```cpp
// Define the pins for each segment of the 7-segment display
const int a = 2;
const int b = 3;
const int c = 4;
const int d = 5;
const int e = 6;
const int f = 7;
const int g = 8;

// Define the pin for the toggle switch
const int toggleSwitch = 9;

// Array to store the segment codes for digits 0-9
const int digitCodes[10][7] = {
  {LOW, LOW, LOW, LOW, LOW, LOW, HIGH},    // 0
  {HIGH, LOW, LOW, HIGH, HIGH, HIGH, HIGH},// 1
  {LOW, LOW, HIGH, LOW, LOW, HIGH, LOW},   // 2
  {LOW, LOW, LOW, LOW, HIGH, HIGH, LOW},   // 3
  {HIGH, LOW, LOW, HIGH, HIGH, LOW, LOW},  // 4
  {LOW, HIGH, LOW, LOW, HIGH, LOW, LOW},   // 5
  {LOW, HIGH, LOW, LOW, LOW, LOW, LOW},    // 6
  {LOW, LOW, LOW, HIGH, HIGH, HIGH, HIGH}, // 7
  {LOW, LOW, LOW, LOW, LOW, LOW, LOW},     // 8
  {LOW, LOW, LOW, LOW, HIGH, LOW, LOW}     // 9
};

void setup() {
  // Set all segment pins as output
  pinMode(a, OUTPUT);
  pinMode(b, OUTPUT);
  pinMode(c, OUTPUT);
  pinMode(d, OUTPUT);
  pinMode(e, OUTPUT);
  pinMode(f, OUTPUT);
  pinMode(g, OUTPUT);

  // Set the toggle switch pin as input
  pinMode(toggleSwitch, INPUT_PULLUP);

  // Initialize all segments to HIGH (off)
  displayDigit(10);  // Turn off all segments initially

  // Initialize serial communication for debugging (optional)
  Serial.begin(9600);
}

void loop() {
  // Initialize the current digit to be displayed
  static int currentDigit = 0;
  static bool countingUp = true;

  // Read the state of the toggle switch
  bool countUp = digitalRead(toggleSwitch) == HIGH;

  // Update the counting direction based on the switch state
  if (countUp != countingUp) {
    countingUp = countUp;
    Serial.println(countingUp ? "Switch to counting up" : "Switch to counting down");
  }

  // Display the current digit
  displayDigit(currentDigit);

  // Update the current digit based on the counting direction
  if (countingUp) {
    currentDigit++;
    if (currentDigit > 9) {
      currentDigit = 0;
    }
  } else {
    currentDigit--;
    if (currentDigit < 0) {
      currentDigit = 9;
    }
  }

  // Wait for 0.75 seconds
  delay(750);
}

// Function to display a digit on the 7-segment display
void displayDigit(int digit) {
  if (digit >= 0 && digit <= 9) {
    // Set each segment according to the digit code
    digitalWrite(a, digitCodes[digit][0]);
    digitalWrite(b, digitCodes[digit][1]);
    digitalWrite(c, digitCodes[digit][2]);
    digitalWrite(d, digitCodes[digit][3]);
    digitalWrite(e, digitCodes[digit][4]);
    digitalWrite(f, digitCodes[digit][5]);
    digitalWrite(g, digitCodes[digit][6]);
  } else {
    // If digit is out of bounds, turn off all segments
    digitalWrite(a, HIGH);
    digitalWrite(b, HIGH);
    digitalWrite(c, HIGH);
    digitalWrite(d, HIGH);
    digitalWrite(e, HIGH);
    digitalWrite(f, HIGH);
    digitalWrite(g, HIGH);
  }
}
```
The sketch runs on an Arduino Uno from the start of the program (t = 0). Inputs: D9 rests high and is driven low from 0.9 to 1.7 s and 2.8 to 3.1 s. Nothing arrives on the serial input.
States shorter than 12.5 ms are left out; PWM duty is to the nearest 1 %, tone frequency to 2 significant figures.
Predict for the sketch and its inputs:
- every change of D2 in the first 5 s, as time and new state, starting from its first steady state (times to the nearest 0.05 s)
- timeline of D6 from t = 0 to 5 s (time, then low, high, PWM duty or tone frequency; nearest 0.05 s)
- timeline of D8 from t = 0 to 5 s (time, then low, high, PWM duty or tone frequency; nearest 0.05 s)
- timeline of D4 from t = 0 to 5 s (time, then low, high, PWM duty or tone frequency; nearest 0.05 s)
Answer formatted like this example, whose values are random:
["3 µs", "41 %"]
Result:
["0 s low; 0.75 s high; 1.5 s low; 2.25 s high; 3 s low; 3.75 s high; 4.5 s low", "0 s low; 0.75 s high; 1.5 s low; 2.25 s high; 3 s low; 3.75 s high; 4.5 s low", "0 s high; 1.5 s low; 2.25 s high; 3 s low; 3.75 s high; 4.5 s low", "0 s low; 1.5 s high; 2.25 s low; 3 s high; 3.75 s low; 4.5 s high"]
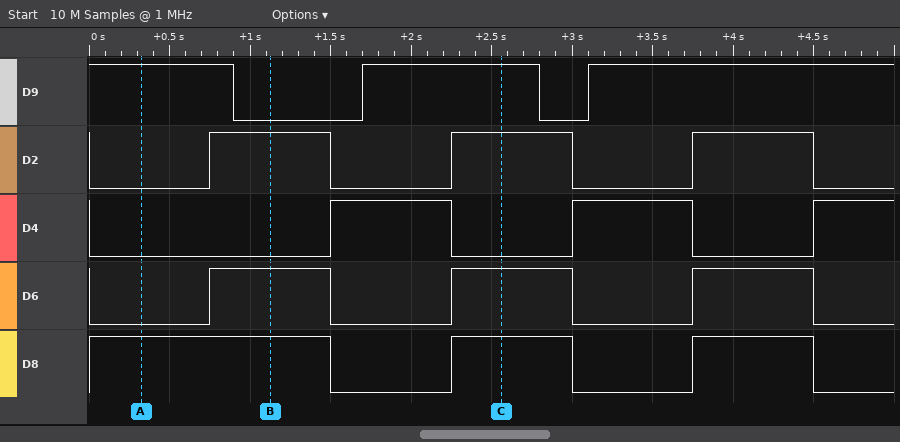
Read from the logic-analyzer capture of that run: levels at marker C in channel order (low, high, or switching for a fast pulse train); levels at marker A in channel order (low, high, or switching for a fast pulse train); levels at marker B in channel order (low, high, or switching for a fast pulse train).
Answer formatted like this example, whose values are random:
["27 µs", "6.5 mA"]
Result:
["D9 high, D2 high, D4 low, D6 high, D8 high", "D9 high, D2 low, D4 low, D6 low, D8 high", "D9 low, D2 high, D4 low, D6 high, D8 high"]
